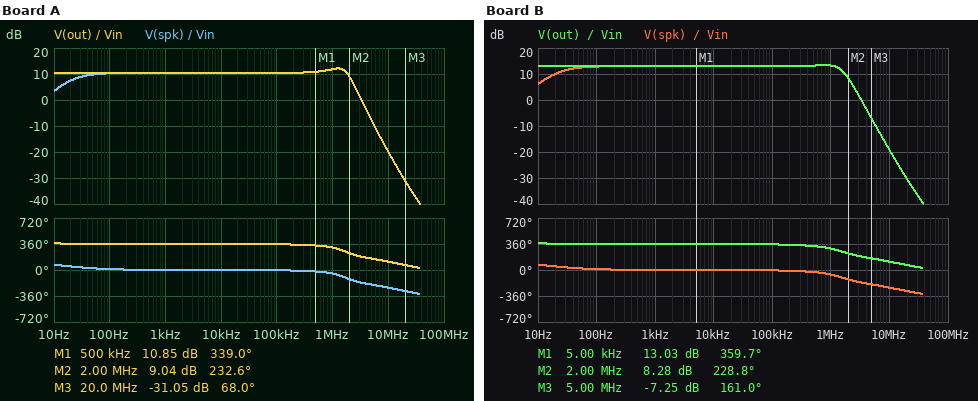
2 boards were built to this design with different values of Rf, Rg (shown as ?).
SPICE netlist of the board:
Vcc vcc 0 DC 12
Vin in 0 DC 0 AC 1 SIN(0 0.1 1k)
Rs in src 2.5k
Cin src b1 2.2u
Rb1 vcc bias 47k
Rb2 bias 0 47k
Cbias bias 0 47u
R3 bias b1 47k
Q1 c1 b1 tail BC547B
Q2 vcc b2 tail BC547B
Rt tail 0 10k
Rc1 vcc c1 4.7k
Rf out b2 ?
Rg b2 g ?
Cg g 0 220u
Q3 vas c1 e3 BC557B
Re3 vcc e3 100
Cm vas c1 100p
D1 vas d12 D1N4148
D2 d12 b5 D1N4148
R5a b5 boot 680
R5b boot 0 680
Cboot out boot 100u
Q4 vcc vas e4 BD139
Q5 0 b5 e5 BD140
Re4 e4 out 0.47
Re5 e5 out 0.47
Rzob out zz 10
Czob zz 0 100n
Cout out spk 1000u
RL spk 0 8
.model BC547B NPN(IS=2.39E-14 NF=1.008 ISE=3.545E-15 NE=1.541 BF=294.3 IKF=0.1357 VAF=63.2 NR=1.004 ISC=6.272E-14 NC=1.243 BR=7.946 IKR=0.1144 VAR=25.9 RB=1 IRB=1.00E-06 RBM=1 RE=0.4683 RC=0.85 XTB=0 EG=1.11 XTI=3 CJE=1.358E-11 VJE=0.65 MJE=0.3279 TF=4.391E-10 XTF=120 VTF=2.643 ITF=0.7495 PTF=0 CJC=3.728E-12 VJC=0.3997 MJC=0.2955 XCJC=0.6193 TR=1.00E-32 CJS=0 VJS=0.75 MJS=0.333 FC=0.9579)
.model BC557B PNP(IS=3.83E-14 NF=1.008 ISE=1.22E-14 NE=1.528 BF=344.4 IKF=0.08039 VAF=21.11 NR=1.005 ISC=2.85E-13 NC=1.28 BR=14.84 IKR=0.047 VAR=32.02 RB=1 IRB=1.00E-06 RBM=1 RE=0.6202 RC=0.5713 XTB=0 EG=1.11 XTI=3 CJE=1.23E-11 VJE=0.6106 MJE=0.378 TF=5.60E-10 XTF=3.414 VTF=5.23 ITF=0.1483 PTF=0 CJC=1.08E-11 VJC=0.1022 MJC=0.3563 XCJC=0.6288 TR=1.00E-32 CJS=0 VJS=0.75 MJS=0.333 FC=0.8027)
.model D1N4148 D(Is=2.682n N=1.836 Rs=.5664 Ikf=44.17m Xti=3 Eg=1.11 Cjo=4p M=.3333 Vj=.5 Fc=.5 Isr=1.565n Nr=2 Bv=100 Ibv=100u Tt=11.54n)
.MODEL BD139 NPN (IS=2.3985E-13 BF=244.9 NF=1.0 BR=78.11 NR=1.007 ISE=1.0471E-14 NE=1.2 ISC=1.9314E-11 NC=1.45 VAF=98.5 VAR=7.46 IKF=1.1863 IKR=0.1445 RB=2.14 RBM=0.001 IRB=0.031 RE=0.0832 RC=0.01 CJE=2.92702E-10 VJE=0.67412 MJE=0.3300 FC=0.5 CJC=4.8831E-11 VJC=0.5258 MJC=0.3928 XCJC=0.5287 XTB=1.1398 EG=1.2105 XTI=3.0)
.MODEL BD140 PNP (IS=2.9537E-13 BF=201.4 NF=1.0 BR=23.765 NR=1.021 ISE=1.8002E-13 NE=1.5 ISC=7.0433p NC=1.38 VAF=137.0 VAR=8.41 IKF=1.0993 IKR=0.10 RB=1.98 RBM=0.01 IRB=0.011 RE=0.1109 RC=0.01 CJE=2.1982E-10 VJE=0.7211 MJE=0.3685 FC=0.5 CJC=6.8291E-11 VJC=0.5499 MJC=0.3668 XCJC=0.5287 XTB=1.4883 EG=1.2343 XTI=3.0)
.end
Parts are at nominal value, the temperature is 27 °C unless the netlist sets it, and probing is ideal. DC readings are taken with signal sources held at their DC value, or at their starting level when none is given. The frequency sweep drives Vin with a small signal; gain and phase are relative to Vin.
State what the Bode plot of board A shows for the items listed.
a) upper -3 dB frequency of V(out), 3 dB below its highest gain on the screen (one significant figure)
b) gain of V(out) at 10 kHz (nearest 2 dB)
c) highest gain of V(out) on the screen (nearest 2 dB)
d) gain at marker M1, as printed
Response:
2 MHz
10 dB
12 dB
10.85 dB
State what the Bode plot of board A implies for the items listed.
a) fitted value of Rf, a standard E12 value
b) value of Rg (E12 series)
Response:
6.8 kΩ
2.7 kΩ
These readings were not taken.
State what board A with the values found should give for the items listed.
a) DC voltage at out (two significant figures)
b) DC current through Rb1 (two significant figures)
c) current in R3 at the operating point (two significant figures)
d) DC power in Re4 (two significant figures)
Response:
6.0 V
130 µA
760 nA
510 µW
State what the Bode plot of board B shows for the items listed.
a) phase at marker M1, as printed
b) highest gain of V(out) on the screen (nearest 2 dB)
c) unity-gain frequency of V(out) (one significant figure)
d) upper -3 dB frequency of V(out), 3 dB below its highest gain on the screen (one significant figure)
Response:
359.7 deg
14 dB
3 MHz
2 MHz
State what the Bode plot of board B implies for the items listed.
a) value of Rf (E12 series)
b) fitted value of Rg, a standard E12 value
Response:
6.8 kΩ
1.8 kΩ
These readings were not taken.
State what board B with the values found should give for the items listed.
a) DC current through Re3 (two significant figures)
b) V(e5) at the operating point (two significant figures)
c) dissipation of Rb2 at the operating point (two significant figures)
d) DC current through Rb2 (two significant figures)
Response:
3.9 mA
5.9 V
760 µW
130 µA
